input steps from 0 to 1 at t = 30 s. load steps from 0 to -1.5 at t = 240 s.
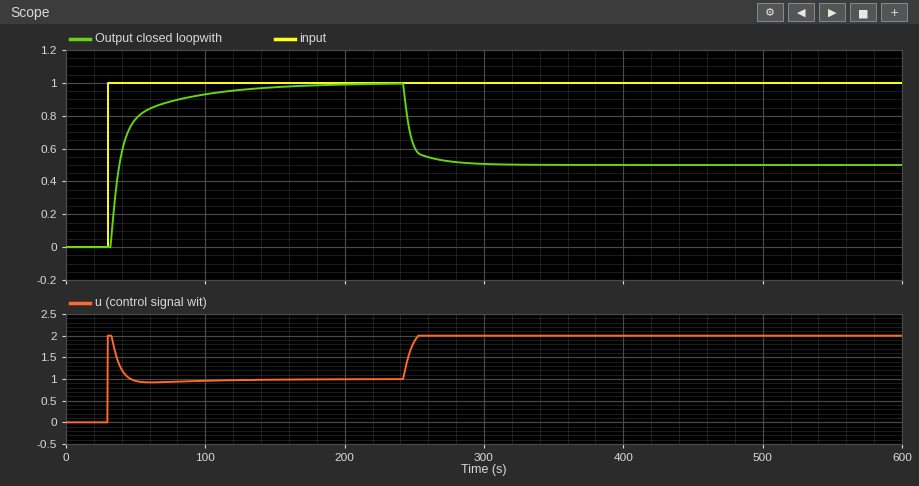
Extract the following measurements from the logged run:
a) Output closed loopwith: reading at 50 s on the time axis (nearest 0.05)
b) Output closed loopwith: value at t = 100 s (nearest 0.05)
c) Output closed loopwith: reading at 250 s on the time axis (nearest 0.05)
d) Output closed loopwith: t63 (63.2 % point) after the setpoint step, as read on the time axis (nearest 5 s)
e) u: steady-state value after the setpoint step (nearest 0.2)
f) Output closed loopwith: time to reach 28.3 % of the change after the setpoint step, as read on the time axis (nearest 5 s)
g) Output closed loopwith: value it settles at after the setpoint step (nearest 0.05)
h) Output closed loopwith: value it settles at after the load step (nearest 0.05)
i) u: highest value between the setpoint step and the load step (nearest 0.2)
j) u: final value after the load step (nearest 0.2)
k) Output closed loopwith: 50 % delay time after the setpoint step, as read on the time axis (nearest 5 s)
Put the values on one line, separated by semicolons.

0.80; 0.95; 0.60; 40 s; 1.0; 35 s; 1.00; 0.50; 2.0; 2.0; 40 s
